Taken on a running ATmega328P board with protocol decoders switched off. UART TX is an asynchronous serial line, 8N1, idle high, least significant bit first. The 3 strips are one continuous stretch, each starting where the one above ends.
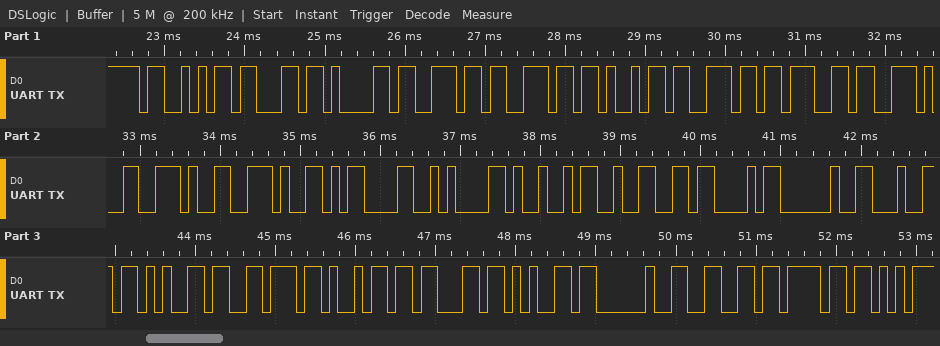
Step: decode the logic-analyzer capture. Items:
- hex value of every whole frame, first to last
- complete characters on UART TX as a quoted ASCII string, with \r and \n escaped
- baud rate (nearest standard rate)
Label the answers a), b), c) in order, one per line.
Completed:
a) 53 63 61 6E 6E 69 6E 67 2E 2E 2E 0D 0A 49 32 43 20 64 65 76 69 63 65 20 66 6F
b) "Scanning...\r\nI2C device fo"
c) 9600 baud
